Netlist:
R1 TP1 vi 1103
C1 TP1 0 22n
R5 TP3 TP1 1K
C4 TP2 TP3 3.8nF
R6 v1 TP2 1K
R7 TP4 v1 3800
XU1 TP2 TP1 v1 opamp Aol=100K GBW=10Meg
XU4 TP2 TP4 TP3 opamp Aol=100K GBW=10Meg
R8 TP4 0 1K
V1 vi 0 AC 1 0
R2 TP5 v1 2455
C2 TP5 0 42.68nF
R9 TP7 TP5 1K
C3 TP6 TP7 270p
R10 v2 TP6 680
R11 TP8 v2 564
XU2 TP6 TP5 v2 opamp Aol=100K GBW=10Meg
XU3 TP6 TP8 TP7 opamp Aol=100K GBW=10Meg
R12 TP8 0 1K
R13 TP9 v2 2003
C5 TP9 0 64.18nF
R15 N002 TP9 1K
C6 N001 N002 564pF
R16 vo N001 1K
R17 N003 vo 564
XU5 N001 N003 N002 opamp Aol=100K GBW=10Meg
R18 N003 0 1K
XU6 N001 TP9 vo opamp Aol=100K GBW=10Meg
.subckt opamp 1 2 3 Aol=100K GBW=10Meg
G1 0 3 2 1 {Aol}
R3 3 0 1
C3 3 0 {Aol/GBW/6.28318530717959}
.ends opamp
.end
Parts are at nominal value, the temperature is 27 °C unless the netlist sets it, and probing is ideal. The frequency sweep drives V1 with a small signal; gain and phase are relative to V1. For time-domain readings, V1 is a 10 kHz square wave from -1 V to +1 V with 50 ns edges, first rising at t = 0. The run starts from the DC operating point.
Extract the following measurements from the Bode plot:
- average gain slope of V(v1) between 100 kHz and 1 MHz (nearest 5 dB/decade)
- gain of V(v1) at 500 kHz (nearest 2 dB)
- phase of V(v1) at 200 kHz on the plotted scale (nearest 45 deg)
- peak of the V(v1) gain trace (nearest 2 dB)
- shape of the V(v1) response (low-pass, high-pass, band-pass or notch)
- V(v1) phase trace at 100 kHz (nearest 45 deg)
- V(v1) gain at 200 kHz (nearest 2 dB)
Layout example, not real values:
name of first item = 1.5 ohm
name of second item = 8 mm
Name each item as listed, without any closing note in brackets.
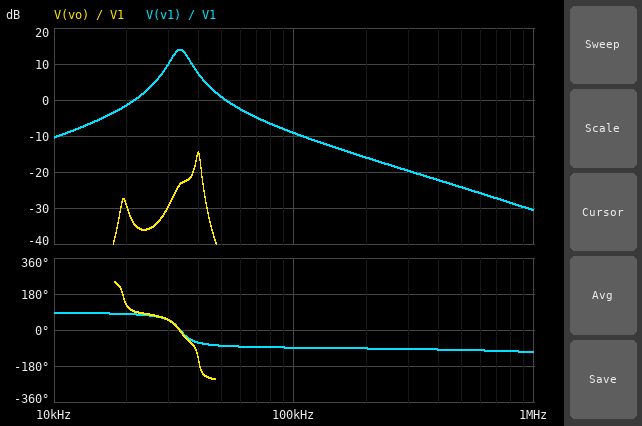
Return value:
average gain slope of V(v1) between 100 kHz and 1 MHz = -20 dB/decade
gain of V(v1) at 500 kHz = -24 dB
phase of V(v1) at 200 kHz on the plotted scale = -90 deg
peak of the V(v1) gain trace = 14 dB
shape of the V(v1) response = band-pass
V(v1) phase trace at 100 kHz = -90 deg
V(v1) gain at 200 kHz = -16 dB
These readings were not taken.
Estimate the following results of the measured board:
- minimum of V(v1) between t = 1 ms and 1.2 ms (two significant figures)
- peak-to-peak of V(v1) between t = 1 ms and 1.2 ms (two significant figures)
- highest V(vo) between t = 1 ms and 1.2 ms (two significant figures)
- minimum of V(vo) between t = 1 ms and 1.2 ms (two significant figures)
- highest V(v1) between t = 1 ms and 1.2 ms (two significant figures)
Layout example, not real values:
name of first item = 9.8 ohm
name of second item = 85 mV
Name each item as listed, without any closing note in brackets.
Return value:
minimum of V(v1) between t = 1 ms and 1.2 ms = -1.9 V
peak-to-peak of V(v1) between t = 1 ms and 1.2 ms = 3.8 V
highest V(vo) between t = 1 ms and 1.2 ms = 16 mV
minimum of V(vo) between t = 1 ms and 1.2 ms = -16 mV
highest V(v1) between t = 1 ms and 1.2 ms = 1.9 V
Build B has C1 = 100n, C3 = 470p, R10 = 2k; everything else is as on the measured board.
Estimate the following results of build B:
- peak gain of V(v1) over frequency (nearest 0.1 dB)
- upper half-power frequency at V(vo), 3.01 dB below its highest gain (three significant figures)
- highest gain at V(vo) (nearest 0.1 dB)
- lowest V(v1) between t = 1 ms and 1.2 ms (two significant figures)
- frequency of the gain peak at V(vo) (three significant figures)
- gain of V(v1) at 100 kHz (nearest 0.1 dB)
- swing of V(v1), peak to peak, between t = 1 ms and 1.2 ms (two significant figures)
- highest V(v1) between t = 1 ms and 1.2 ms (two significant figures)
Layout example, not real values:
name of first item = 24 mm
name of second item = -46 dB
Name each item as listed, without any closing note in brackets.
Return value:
peak gain of V(v1) over frequency = 14.0 dB
upper half-power frequency at V(vo), 3.01 dB below its highest gain = 19.6 kHz
highest gain at V(vo) = 5.3 dB
lowest V(v1) between t = 1 ms and 1.2 ms = -590 mV
frequency of the gain peak at V(vo) = 19.0 kHz
gain of V(v1) at 100 kHz = -23.1 dB
swing of V(v1), peak to peak, between t = 1 ms and 1.2 ms = 1.2 V
highest V(v1) between t = 1 ms and 1.2 ms = 590 mV
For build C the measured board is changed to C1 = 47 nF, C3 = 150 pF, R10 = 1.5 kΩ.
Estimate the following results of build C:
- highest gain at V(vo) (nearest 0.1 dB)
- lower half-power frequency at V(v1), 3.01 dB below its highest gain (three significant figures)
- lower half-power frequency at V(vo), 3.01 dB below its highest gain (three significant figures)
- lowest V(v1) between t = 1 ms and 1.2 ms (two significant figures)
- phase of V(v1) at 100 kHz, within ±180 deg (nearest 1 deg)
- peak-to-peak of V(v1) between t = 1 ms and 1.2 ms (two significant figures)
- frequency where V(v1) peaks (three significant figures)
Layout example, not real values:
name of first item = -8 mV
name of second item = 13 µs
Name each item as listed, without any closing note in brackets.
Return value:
highest gain at V(vo) = -18.1 dB
lower half-power frequency at V(v1), 3.01 dB below its highest gain = 21.6 kHz
lower half-power frequency at V(vo), 3.01 dB below its highest gain = 19.0 kHz
lowest V(v1) between t = 1 ms and 1.2 ms = -760 mV
phase of V(v1) at 100 kHz, within ±180 deg = -90 deg
peak-to-peak of V(v1) between t = 1 ms and 1.2 ms = 1.5 V
frequency where V(v1) peaks = 23.0 kHz
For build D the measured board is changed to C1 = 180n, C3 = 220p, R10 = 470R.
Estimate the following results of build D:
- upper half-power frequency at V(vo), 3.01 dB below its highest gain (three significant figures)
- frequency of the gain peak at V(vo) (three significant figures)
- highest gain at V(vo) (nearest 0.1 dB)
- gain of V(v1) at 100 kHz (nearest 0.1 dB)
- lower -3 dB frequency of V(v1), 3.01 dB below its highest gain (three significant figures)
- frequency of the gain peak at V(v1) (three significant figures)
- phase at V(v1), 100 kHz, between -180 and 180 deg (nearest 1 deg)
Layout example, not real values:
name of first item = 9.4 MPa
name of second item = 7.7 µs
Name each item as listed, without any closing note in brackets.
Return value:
upper half-power frequency at V(vo), 3.01 dB below its highest gain = 20.1 kHz
frequency of the gain peak at V(vo) = 19.4 kHz
highest gain at V(vo) = -41.2 dB
gain of V(v1) at 100 kHz = -28.3 dB
lower -3 dB frequency of V(v1), 3.01 dB below its highest gain = 11.4 kHz
frequency of the gain peak at V(v1) = 11.7 kHz
phase at V(v1), 100 kHz, between -180 and 180 deg = -92 deg
